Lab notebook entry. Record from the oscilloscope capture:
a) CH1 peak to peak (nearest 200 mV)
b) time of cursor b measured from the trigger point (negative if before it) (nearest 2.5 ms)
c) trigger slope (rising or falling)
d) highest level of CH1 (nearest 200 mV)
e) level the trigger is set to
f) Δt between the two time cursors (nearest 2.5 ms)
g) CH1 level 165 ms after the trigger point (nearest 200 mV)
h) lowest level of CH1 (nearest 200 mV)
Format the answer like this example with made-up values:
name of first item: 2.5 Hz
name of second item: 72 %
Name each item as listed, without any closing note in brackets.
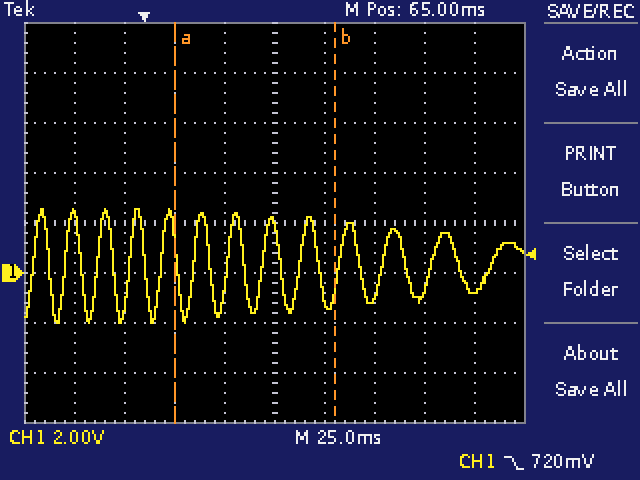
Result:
CH1 peak to peak: 4.6 V
time of cursor b measured from the trigger point (negative if before it): +95.0 ms
trigger slope: falling
highest level of CH1: 2.6 V
level the trigger is set to: 720 mV
Δt between the two time cursors: 80.0 ms
CH1 level 165 ms after the trigger point: -800 mV
lowest level of CH1: -2.0 V
